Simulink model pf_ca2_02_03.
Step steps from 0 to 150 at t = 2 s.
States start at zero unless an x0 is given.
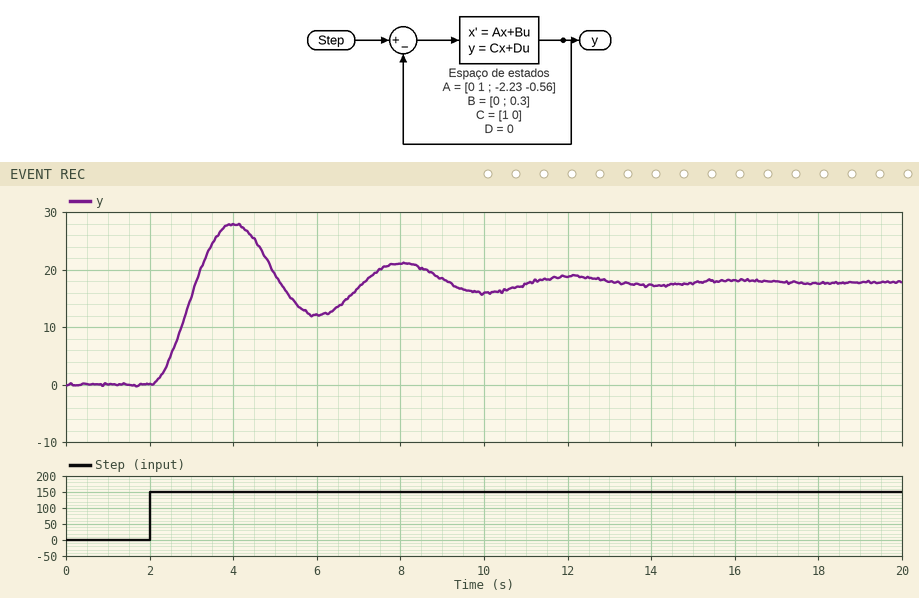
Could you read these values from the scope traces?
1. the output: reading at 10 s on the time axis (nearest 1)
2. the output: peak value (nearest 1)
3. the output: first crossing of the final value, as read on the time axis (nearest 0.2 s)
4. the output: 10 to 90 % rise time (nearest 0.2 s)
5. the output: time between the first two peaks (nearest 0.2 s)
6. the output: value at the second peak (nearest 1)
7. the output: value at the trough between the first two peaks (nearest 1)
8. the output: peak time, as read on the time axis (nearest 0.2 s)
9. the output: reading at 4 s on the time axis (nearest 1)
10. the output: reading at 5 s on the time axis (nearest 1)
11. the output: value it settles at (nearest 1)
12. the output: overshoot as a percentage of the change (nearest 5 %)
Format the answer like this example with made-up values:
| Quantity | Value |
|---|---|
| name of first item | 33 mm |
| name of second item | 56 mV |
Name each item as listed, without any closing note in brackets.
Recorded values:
| Quantity | Value |
|---|---|
| the output: reading at 10 s on the time axis | 16 |
| the output: peak value | 28 |
| the output: first crossing of the final value, as read on the time axis | 3.2 s |
| the output: 10 to 90 % rise time | 0.8 s |
| the output: time between the first two peaks | 4.0 s |
| the output: value at the second peak | 21 |
| the output: value at the trough between the first two peaks | 12 |
| the output: peak time, as read on the time axis | 4.0 s |
| the output: reading at 4 s on the time axis | 28 |
| the output: reading at 5 s on the time axis | 19 |
| the output: value it settles at | 18 |
| the output: overshoot as a percentage of the change | 55 % |
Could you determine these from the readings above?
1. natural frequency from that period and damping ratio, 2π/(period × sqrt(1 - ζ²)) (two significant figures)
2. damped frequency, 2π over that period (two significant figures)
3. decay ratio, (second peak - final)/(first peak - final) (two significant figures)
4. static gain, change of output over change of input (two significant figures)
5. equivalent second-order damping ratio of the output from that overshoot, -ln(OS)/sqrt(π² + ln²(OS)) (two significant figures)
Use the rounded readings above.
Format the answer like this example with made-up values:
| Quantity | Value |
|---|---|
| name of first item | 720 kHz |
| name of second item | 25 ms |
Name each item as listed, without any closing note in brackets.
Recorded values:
| Quantity | Value |
|---|---|
| natural frequency from that period and damping ratio, 2π/(period × sqrt(1 - ζ²)) | 1.6 rad/s |
| damped frequency, 2π over that period | 1.6 rad/s |
| decay ratio, (second peak - final)/(first peak - final) | 0.30 |
| static gain, change of output over change of input | 0.12 |
| equivalent second-order damping ratio of the output from that overshoot, -ln(OS)/sqrt(π² + ln²(OS)) | 0.19 |
